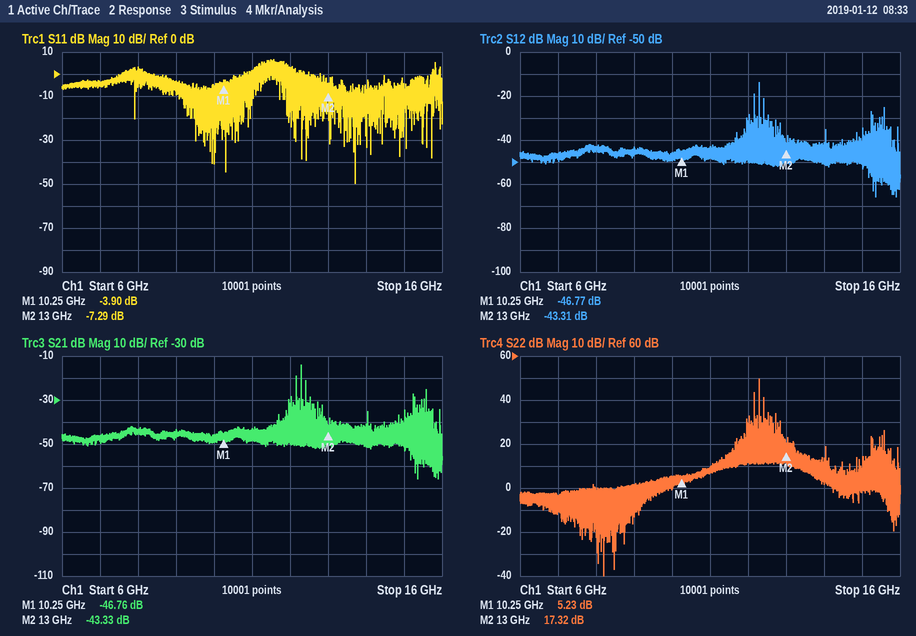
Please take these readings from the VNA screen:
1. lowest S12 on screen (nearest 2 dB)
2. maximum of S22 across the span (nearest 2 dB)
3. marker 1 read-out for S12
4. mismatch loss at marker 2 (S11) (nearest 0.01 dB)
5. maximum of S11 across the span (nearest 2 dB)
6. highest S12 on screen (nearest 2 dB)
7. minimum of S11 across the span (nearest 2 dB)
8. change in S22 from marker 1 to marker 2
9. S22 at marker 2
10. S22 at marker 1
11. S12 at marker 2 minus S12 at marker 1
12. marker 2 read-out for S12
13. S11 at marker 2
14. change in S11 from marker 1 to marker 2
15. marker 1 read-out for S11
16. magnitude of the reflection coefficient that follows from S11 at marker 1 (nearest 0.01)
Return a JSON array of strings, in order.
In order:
["-66 dB", "50 dB", "-46.77 dB", "0.90 dB", "6 dB", "-14 dB", "-50 dB", "12.09 dB", "17.32 dB", "5.23 dB", "3.46 dB", "-43.31 dB", "-7.29 dB", "-3.39 dB", "-3.90 dB", "0.64"]
